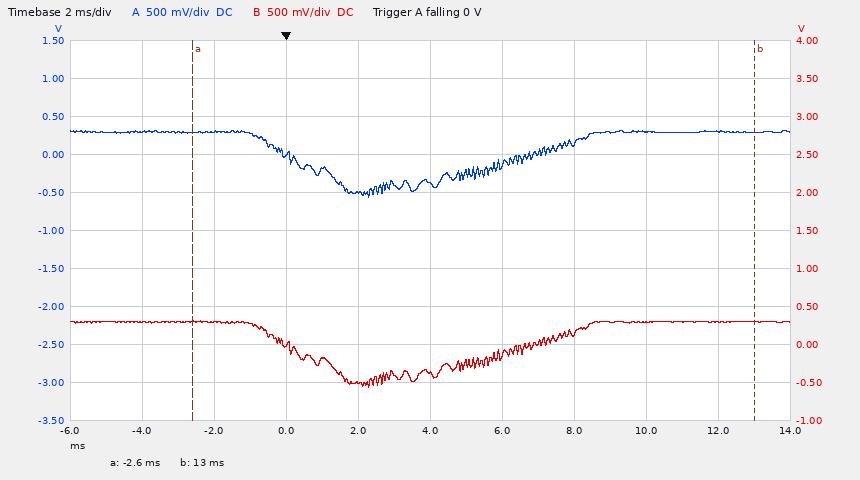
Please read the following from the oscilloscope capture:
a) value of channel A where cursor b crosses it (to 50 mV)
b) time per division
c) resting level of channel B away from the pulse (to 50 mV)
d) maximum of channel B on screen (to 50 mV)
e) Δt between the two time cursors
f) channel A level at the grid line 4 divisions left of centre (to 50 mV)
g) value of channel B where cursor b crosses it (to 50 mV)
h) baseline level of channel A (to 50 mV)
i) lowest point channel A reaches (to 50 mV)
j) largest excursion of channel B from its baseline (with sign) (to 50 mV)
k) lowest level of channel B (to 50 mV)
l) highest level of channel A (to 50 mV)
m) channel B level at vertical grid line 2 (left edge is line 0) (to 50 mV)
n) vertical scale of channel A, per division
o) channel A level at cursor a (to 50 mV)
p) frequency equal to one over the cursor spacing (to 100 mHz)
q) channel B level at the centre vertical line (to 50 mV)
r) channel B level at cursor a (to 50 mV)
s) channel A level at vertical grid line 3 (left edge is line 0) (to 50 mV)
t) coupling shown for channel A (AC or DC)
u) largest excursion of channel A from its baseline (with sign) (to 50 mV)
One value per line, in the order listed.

300 mV
2 ms
300 mV
300 mV
15.6 ms
300 mV
300 mV
300 mV
-550 mV
-850 mV
-550 mV
300 mV
300 mV
500 mV
300 mV
64.1 Hz
-400 mV
300 mV
0 mV
DC
-850 mV
